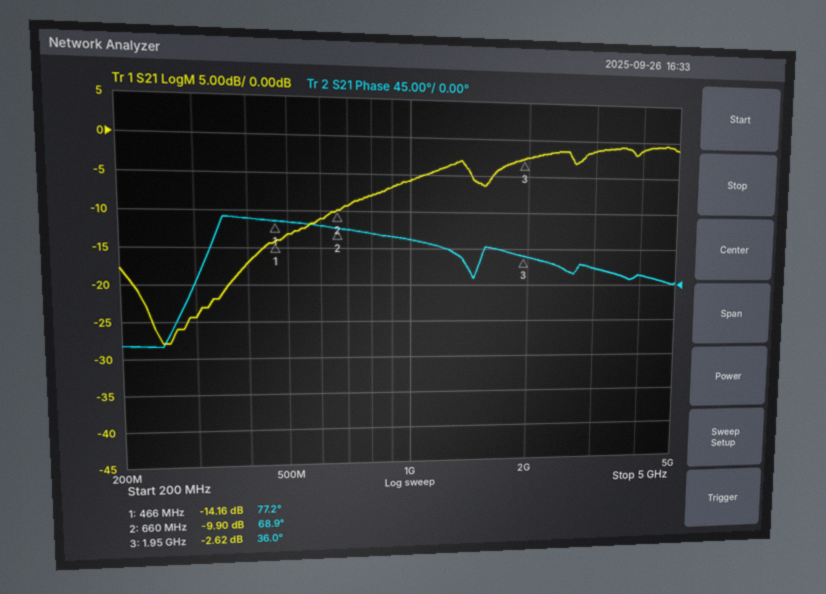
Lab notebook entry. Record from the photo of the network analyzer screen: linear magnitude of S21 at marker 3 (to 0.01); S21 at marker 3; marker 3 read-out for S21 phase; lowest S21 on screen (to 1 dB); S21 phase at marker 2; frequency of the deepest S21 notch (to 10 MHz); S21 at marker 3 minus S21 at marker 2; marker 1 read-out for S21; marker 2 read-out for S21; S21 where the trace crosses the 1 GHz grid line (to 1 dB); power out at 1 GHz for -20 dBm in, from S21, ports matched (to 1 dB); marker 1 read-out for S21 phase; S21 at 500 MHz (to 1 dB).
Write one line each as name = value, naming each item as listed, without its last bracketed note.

linear magnitude of S21 at marker 3 = 0.74
S21 at marker 3 = -2.62 dB
marker 3 read-out for S21 phase = 36.0°
lowest S21 on screen = -28 dB
S21 phase at marker 2 = 68.9°
frequency of the deepest S21 notch = 250 MHz
S21 at marker 3 minus S21 at marker 2 = 7.28 dB
marker 1 read-out for S21 = -14.16 dB
marker 2 read-out for S21 = -9.90 dB
S21 where the trace crosses the 1 GHz grid line = -6 dB
power out at 1 GHz for -20 dBm in, from S21, ports matched = -26 dBm
marker 1 read-out for S21 phase = 77.2°
S21 at 500 MHz = -13 dB
